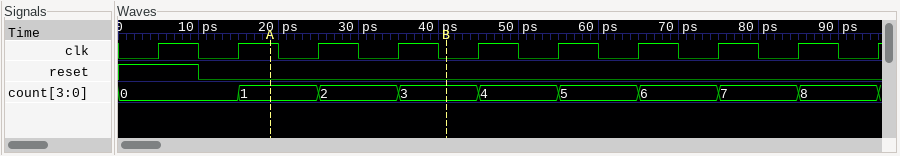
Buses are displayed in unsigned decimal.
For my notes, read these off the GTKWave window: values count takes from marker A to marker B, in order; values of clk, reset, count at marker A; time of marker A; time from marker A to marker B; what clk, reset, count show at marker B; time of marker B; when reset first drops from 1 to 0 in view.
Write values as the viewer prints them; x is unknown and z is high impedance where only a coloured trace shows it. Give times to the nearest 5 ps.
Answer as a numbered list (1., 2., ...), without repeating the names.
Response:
1. 1, 2, 3
2. clk=1, reset=0, count=1
3. 20 ps
4. 20 ps
5. clk=0, reset=0, count=3
6. 40 ps
7. 10 ps
